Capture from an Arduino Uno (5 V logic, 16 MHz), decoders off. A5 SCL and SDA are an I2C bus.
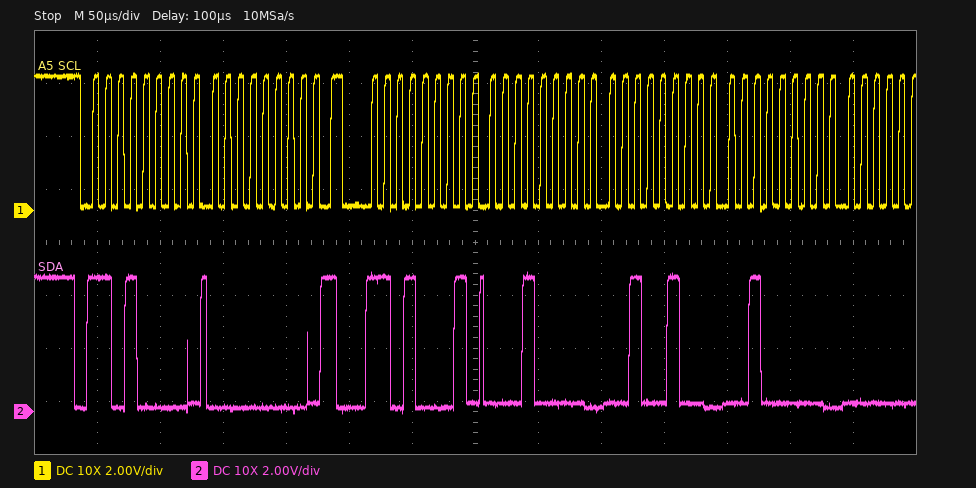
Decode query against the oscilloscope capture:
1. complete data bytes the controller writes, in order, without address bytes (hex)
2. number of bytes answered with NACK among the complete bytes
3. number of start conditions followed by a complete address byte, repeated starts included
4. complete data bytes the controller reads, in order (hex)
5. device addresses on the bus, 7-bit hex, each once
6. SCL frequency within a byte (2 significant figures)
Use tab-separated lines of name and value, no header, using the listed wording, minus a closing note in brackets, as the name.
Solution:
complete data bytes the controller writes, in order, without address bytes	00
number of bytes answered with NACK among the complete bytes	0
number of start conditions followed by a complete address byte, repeated starts included	2
complete data bytes the controller reads, in order	10 24 20
device addresses on the bus, 7-bit hex, each once	0x68
SCL frequency within a byte	100 kHz
